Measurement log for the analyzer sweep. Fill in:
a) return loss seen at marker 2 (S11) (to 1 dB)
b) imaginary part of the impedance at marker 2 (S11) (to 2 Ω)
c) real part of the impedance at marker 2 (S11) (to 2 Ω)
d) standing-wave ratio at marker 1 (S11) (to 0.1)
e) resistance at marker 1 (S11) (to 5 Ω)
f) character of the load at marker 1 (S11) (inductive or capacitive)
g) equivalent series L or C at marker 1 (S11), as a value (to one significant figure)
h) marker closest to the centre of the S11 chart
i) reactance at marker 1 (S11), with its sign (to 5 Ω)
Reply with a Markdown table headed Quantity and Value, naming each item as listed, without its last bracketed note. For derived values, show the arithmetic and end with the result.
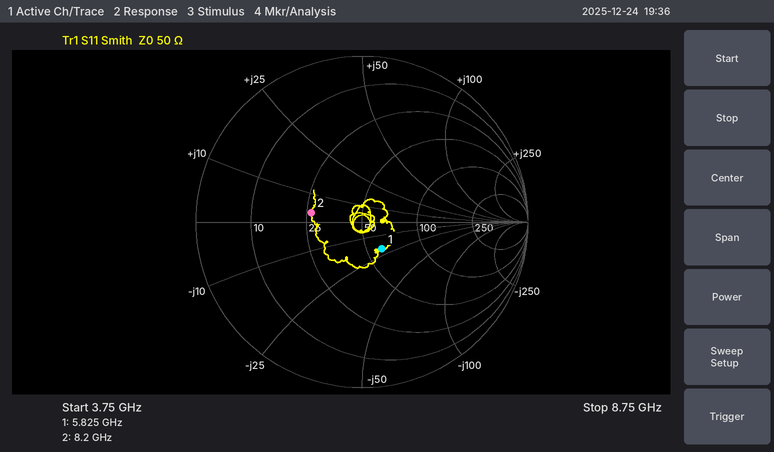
| Quantity | Value |
|---|---|
| return loss seen at marker 2 (S11) | 10 dB |
| imaginary part of the impedance at marker 2 (S11) | +4 Ω |
| real part of the impedance at marker 2 (S11) | 26 Ω |
| standing-wave ratio at marker 1 (S11) | 1.5 |
| resistance at marker 1 (S11) | 60 Ω |
| character of the load at marker 1 (S11) | capacitive |
| equivalent series L or C at marker 1 (S11), as a value | C = 1/(2π × 5.825 GHz × 20 Ω) ≈ 1 pF |
| marker closest to the centre of the S11 chart | marker 1 |
| reactance at marker 1 (S11), with its sign | -20 Ω |
